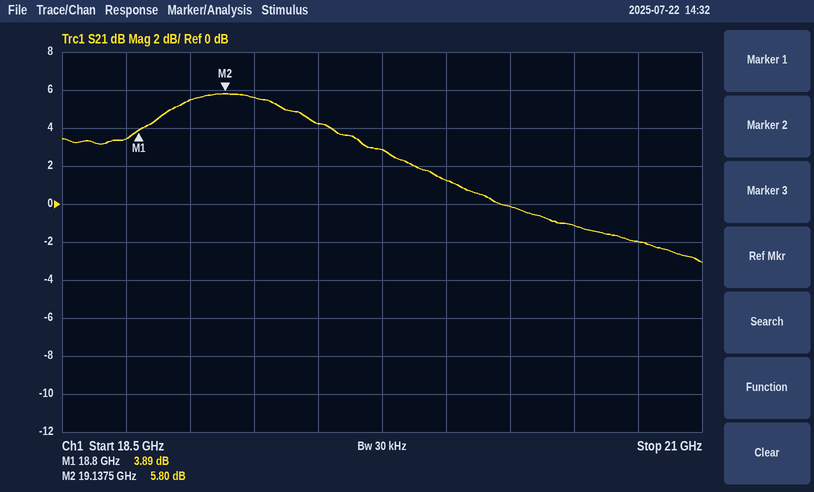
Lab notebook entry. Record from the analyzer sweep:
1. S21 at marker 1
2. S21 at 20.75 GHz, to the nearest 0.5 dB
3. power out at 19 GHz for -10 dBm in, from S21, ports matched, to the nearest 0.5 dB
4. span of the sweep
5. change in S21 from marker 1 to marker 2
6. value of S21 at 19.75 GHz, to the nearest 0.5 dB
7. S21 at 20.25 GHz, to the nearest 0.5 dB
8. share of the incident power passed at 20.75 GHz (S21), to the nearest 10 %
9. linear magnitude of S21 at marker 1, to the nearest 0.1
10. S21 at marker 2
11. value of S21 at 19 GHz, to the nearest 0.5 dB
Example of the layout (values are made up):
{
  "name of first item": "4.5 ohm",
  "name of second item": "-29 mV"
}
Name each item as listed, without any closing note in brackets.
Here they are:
{
  "S21 at marker 1": "3.89 dB",
  "S21 at 20.75 GHz, to the nearest 0.5 dB": "-2.0 dB",
  "power out at 19 GHz for -10 dBm in, from S21, ports matched, to the nearest 0.5 dB": "-4.5 dBm",
  "span of the sweep": "2.5 GHz",
  "change in S21 from marker 1 to marker 2": "1.91 dB",
  "value of S21 at 19.75 GHz, to the nearest 0.5 dB": "3.0 dB",
  "S21 at 20.25 GHz, to the nearest 0.5 dB": "0.0 dB",
  "share of the incident power passed at 20.75 GHz (S21), to the nearest 10 %": "60 %",
  "linear magnitude of S21 at marker 1, to the nearest 0.1": "1.6",
  "S21 at marker 2": "5.80 dB",
  "value of S21 at 19 GHz, to the nearest 0.5 dB": "5.5 dB"
}
